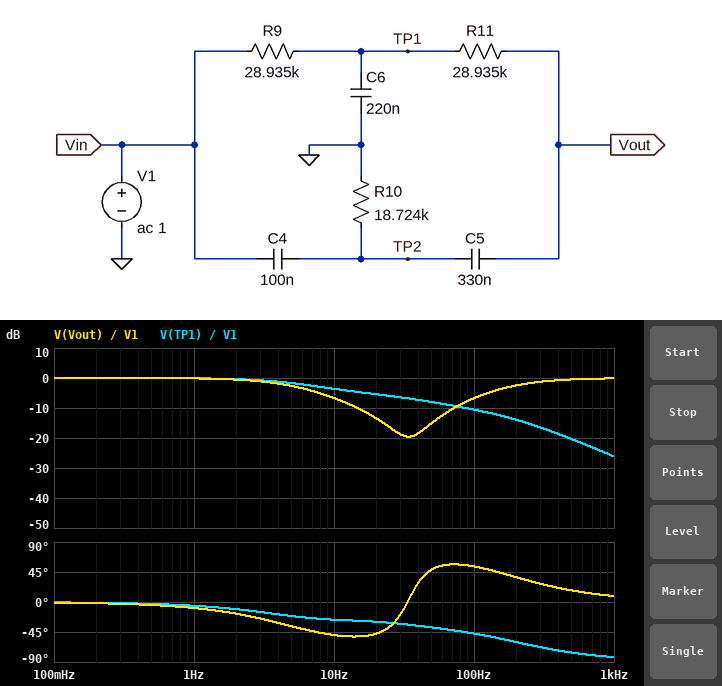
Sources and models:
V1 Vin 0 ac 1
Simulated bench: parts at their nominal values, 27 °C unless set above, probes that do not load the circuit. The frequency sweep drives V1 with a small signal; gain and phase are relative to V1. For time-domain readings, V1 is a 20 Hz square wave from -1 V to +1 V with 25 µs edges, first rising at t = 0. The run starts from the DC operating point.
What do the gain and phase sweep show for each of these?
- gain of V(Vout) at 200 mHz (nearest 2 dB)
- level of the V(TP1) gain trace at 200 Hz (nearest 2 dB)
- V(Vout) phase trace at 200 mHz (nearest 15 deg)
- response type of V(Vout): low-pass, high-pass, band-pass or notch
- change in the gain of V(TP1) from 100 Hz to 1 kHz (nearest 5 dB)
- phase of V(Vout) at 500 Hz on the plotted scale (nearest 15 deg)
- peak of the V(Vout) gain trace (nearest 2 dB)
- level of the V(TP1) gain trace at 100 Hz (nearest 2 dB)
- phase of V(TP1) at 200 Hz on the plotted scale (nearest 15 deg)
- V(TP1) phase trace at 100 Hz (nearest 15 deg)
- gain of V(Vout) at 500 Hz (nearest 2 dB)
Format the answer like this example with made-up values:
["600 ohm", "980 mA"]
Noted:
["0 dB", "-14 dB", "0 deg", "notch", "-15 dB", "15 deg", "0 dB", "-10 dB", "-60 deg", "-45 deg", "0 dB"]
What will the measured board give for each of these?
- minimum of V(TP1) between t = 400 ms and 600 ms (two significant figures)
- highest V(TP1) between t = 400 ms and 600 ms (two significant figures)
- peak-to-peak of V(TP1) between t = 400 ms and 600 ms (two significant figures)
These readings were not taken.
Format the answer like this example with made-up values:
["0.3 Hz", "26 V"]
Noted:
["-700 mV", "700 mV", "1.4 V"]
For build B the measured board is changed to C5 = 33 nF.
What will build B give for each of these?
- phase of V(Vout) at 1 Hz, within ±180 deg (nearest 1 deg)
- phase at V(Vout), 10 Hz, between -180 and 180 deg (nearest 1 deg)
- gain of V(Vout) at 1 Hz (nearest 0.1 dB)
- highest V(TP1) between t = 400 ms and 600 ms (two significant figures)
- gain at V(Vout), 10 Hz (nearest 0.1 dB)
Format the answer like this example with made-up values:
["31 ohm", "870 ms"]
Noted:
["-3 deg", "-28 deg", "0 dB", "930 mV", "-1.0 dB"]
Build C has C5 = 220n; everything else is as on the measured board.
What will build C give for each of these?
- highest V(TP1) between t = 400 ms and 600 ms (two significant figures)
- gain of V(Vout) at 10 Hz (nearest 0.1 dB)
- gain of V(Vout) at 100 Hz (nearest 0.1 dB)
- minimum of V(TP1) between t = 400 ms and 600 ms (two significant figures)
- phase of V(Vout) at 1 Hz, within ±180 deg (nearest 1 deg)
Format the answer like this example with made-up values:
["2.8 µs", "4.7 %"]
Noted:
["740 mV", "-4.7 dB", "-7.2 dB", "-740 mV", "-7 deg"]
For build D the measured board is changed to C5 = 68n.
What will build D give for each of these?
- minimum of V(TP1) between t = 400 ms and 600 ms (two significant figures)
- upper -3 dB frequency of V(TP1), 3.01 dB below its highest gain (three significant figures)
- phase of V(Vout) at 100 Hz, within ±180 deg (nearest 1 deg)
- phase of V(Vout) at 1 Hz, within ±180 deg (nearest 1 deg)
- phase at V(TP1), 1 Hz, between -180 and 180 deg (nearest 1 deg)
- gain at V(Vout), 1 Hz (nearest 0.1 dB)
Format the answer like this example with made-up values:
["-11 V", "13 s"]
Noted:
["-880 mV", "17.0 Hz", "74 deg", "-4 deg", "-3 deg", "0 dB"]
